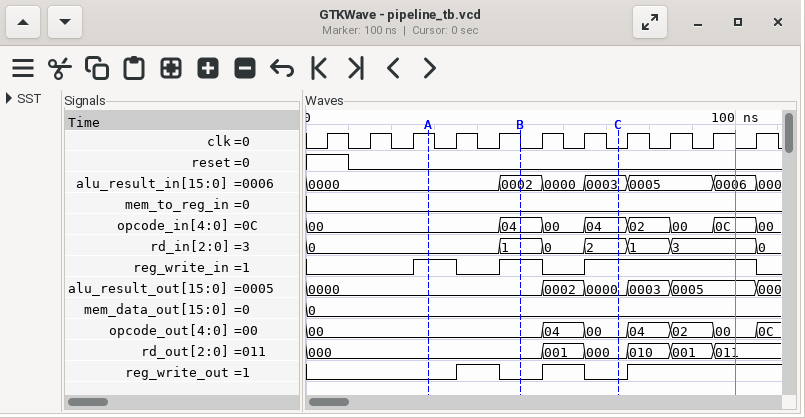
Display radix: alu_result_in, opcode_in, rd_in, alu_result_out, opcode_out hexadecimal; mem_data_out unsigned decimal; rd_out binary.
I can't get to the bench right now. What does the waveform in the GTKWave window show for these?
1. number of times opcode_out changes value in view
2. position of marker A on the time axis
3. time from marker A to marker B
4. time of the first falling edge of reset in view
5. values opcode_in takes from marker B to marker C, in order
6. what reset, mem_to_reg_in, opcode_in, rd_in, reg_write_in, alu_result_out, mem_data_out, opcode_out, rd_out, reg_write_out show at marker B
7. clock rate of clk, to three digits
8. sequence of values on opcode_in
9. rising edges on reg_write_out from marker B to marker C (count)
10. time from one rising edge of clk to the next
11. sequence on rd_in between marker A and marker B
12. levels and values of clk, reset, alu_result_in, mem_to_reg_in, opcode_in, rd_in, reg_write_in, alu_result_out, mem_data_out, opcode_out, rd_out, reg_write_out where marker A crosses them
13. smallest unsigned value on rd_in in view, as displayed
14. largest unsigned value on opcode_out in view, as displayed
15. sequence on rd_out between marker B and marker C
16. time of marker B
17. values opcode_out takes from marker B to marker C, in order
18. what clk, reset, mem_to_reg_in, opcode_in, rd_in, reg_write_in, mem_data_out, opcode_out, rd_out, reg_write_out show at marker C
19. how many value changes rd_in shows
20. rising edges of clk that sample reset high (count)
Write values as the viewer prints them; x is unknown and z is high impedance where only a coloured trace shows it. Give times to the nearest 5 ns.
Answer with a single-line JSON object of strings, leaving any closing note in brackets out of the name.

{"number of times opcode_out changes value in view": "6", "position of marker A on the time axis": "30 ns", "time from marker A to marker B": "20 ns", "time of the first falling edge of reset in view": "10 ns", "values opcode_in takes from marker B to marker C, in order": "04, 00, 04", "what reset, mem_to_reg_in, opcode_in, rd_in, reg_write_in, alu_result_out, mem_data_out, opcode_out, rd_out, reg_write_out show at marker B": "reset=0, mem_to_reg_in=0, opcode_in=04, rd_in=1, reg_write_in=1, alu_result_out=0000, mem_data_out=0, opcode_out=00, rd_out=000, reg_write_out=0", "clock rate of clk, to three digits": "100 MHz", "sequence of values on opcode_in": "00, 04, 00, 04, 02, 00, 0C, 00", "rising edges on reg_write_out from marker B to marker C": "1", "time from one rising edge of clk to the next": "10 ns", "sequence on rd_in between marker A and marker B": "0, 1", "levels and values of clk, reset, alu_result_in, mem_to_reg_in, opcode_in, rd_in, reg_write_in, alu_result_out, mem_data_out, opcode_out, rd_out, reg_write_out where marker A crosses them": "clk=1, reset=0, alu_result_in=0000, mem_to_reg_in=0, opcode_in=00, rd_in=0, reg_write_in=1, alu_result_out=0000, mem_data_out=0, opcode_out=00, rd_out=000, reg_write_out=0", "smallest unsigned value on rd_in in view, as displayed": "0", "largest unsigned value on opcode_out in view, as displayed": "0C", "sequence on rd_out between marker B and marker C": "000, 001, 000", "time of marker B": "50 ns", "values opcode_out takes from marker B to marker C, in order": "00, 04, 00", "what clk, reset, mem_to_reg_in, opcode_in, rd_in, reg_write_in, mem_data_out, opcode_out, rd_out, reg_write_out show at marker C": "clk=0, reset=0, mem_to_reg_in=0, opcode_in=04, rd_in=2, reg_write_in=1, mem_data_out=0, opcode_out=00, rd_out=000, reg_write_out=0", "how many value changes rd_in shows": "6", "rising edges of clk that sample reset high": "1"}
